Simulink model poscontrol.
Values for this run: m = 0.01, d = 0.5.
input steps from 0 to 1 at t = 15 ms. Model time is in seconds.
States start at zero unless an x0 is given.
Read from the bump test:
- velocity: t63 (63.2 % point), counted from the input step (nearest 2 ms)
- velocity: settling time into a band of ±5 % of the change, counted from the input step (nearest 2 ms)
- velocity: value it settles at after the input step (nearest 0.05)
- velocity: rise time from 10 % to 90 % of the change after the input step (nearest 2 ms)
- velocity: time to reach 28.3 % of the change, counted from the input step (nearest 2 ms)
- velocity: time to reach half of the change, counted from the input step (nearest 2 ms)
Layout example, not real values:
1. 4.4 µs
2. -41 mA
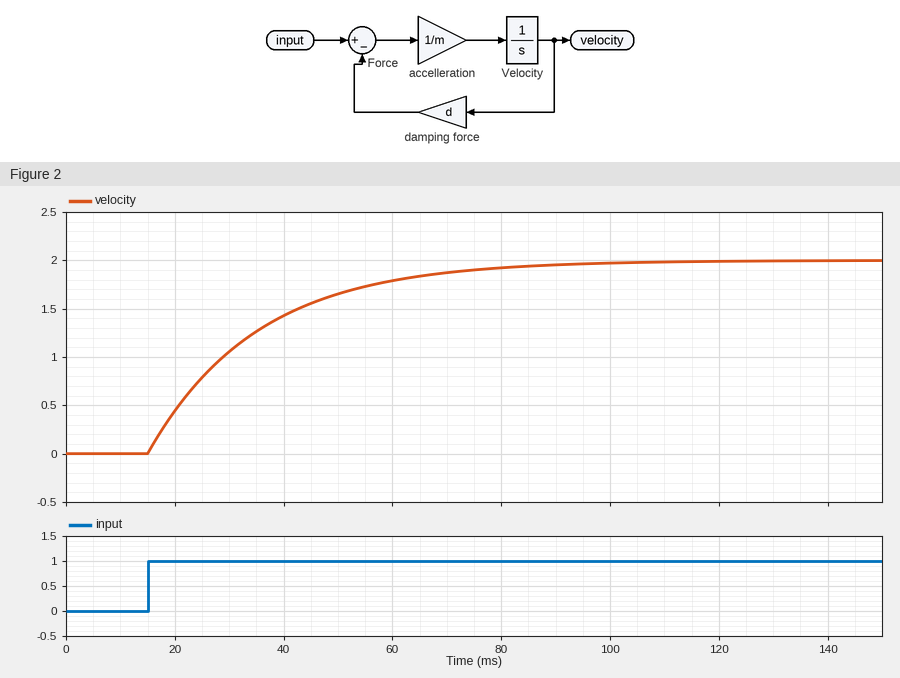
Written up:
1. 20 ms
2. 60 ms
3. 2.00
4. 44 ms
5. 6 ms
6. 14 ms
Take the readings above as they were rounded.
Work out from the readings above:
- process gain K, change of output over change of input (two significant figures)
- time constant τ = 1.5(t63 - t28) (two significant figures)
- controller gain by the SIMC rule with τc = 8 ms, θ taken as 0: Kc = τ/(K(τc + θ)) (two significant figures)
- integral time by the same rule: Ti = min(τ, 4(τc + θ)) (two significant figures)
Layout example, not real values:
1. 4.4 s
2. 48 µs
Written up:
1. 2.0
2. 21 ms
3. 1.3
4. 21 ms
